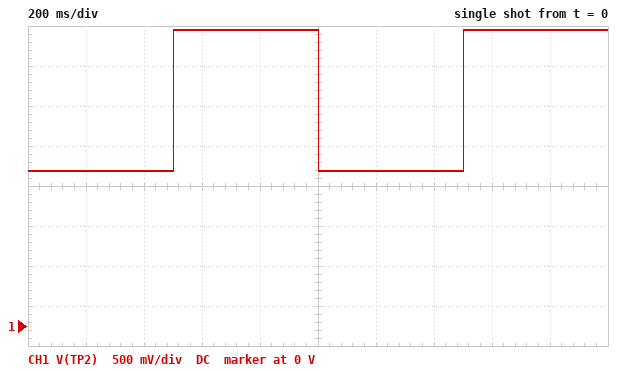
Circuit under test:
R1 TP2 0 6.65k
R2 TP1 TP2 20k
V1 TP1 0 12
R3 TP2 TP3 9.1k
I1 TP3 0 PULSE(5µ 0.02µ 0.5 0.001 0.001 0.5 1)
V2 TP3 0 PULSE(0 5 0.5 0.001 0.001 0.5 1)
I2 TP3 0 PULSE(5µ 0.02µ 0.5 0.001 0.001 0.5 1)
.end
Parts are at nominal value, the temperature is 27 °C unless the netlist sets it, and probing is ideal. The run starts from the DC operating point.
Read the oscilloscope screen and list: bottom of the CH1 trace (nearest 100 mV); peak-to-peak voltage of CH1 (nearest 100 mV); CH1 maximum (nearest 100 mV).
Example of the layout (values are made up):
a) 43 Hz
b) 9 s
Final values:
a) 1.9 V
b) 1.8 V
c) 3.7 V
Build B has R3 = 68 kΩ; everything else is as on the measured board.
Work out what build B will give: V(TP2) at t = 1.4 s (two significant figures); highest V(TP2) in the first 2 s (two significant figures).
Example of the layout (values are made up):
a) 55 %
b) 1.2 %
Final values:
a) 2.8 V
b) 3.1 V
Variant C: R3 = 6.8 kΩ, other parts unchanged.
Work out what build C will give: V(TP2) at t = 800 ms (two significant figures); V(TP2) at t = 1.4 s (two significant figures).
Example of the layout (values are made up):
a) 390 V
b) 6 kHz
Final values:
a) 3.8 V
b) 1.7 V
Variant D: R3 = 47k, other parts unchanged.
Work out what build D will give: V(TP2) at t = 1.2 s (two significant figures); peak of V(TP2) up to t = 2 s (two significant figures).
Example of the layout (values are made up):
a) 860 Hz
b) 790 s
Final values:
a) 2.7 V
b) 3.2 V
